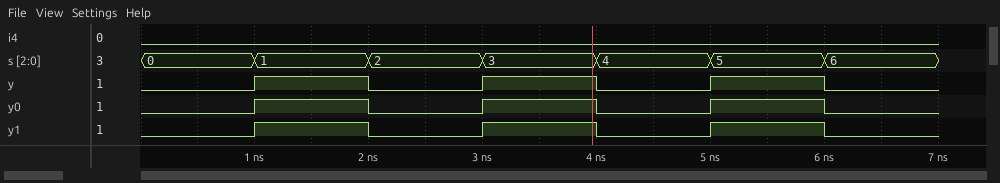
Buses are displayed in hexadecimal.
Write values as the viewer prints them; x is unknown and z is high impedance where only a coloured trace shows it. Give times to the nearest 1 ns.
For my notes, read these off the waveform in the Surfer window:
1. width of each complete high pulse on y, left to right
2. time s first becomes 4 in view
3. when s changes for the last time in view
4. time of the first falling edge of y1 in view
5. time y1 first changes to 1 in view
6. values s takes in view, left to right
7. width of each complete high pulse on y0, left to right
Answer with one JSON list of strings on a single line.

["1 ns, 1 ns, 1 ns", "4 ns", "6 ns", "2 ns", "1 ns", "0, 1, 2, 3, 4, 5, 6", "1 ns, 1 ns, 1 ns"]
